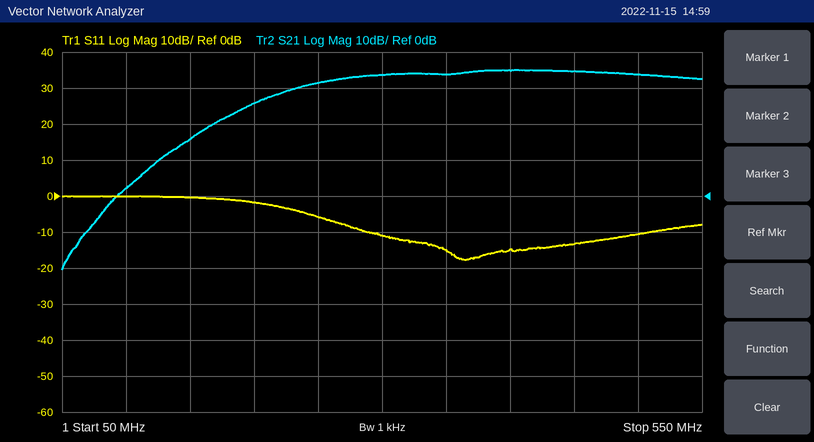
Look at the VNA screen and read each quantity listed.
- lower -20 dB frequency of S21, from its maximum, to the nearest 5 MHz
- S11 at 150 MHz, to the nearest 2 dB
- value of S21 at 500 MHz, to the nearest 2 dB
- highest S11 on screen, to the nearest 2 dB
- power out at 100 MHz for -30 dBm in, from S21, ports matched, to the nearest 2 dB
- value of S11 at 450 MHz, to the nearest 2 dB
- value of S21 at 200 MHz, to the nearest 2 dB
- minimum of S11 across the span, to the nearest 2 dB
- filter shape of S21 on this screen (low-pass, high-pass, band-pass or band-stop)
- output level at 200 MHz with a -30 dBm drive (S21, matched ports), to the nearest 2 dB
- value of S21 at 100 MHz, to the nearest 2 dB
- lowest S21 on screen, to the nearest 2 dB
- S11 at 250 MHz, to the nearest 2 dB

145 MHz
0 dB
34 dB
0 dB
-28 dBm
-14 dB
26 dB
-18 dB
high-pass
-4 dBm
2 dB
-20 dB
-6 dB
